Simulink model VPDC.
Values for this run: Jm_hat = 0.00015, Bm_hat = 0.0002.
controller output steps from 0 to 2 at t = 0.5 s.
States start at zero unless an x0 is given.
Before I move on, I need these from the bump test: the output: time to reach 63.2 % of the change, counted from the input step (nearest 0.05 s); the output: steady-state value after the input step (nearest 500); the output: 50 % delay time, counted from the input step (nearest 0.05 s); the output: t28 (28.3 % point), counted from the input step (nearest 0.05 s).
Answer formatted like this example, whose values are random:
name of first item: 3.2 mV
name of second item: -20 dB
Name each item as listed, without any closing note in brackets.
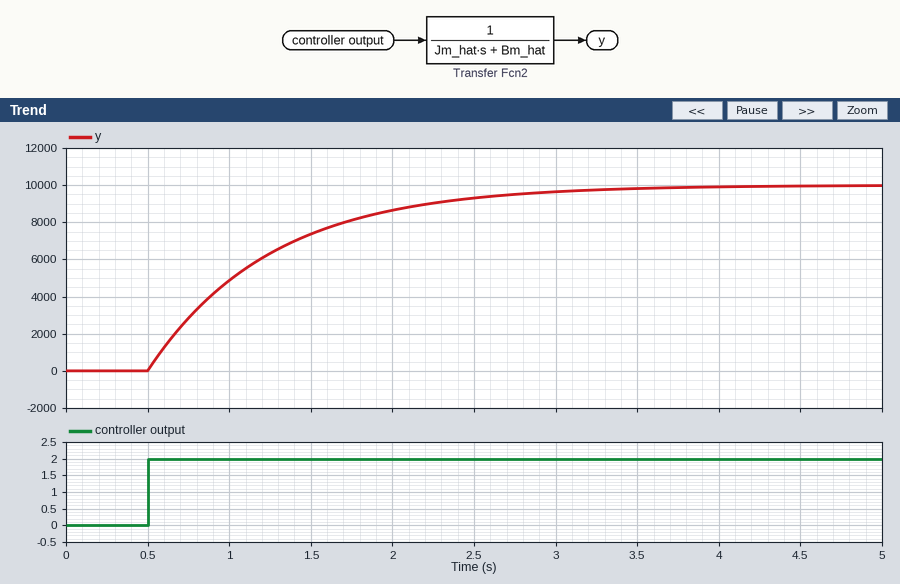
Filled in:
the output: time to reach 63.2 % of the change, counted from the input step: 0.75 s
the output: steady-state value after the input step: 10000
the output: 50 % delay time, counted from the input step: 0.50 s
the output: t28 (28.3 % point), counted from the input step: 0.25 s
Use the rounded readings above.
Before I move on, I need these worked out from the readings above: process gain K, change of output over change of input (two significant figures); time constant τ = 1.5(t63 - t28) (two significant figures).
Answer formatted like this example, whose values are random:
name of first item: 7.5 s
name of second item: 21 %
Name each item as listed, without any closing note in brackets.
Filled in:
process gain K, change of output over change of input: 5000
time constant τ = 1.5(t63 - t28): 0.75 s
